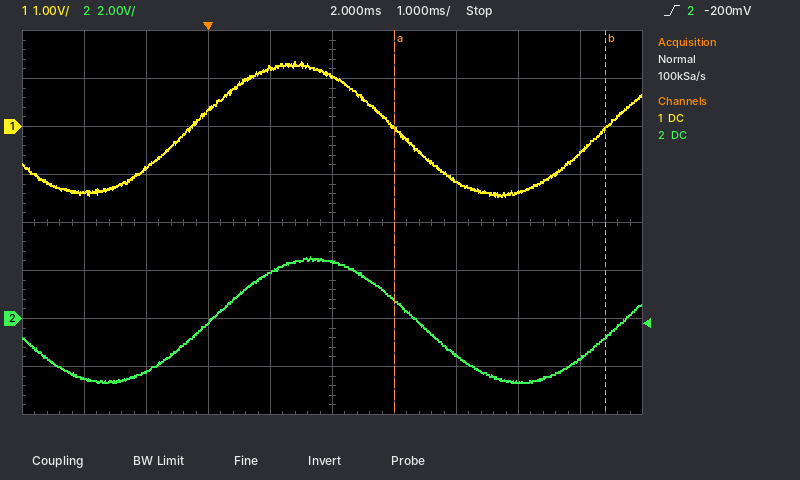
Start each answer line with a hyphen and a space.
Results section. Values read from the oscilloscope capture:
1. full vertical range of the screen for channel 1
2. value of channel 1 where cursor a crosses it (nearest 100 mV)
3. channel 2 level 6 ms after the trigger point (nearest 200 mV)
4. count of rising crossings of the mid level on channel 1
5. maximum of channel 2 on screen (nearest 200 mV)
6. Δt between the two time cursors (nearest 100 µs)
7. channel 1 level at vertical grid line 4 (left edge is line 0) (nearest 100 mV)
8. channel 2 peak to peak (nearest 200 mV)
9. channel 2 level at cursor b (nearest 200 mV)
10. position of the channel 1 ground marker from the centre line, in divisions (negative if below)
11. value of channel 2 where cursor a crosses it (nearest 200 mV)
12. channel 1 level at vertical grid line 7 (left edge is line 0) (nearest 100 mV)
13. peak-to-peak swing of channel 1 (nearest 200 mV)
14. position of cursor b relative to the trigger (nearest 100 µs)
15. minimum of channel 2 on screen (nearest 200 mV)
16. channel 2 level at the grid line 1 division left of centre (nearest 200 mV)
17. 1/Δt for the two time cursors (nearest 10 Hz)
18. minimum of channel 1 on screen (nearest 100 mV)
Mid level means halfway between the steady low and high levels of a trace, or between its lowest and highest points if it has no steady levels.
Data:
- 8 V
- 0.0 V
- -1.6 V
- 2
- 2.6 V
- 3.4 ms
- 1.2 V
- 5.2 V
- -800 mV
- +2.0 div
- 800 mV
- -1.1 V
- 2.8 V
- +6.4 ms
- -2.6 V
- 2.0 V
- 290 Hz
- -1.5 V
